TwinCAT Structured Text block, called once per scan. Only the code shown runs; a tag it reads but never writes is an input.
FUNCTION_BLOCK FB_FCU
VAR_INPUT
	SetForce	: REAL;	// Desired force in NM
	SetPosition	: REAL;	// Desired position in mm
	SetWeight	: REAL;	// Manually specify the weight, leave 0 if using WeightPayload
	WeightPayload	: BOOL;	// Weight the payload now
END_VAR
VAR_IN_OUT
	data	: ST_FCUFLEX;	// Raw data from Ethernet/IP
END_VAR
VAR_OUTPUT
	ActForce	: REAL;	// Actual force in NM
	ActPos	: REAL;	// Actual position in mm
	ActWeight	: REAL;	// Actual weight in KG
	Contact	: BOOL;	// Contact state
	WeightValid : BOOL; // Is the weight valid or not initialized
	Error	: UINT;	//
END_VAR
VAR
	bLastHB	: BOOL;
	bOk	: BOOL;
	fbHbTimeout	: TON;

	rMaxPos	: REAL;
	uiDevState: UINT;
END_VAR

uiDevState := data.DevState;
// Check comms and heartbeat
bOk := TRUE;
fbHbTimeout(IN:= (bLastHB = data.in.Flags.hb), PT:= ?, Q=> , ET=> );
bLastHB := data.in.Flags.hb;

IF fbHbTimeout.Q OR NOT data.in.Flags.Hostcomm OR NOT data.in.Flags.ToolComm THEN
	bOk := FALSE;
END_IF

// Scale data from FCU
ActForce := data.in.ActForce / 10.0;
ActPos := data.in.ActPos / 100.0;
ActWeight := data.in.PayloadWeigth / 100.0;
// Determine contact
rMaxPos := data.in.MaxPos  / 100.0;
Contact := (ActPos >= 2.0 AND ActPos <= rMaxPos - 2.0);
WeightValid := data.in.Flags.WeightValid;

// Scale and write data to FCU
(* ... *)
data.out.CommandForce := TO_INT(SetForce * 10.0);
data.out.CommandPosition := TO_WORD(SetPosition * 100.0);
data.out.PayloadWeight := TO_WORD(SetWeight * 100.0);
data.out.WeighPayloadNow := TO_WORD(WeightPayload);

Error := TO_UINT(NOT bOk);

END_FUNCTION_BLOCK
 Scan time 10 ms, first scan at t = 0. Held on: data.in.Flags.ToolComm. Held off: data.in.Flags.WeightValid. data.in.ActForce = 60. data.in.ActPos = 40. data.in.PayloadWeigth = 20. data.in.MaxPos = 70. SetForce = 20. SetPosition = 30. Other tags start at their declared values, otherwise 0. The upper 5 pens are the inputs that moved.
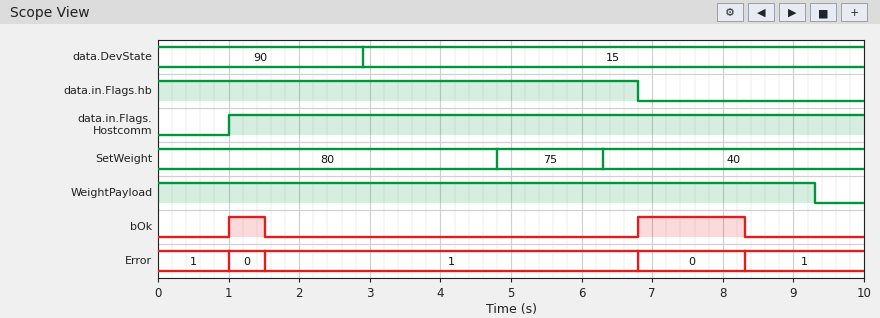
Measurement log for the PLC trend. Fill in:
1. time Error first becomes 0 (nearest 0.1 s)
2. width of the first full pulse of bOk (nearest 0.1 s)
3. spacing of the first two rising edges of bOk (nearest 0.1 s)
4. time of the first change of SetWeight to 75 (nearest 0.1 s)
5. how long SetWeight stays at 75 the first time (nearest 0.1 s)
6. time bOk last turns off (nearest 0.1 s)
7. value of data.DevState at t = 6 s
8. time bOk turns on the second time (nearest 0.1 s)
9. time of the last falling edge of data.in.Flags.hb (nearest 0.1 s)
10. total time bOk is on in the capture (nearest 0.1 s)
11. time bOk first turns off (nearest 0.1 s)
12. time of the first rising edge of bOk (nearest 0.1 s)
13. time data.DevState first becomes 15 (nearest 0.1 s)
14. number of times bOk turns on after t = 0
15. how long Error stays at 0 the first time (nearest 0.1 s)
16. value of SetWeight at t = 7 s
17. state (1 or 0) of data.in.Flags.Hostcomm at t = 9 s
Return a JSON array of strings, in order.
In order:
["1.0 s", "0.5 s", "5.8 s", "4.8 s", "1.5 s", "8.3 s", "15", "6.8 s", "6.8 s", "2.0 s", "1.5 s", "1.0 s", "2.9 s", "2", "0.5 s", "40", "1"]
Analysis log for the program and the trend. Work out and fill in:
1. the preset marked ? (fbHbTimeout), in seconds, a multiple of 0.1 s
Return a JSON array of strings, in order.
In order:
["1.5 s"]
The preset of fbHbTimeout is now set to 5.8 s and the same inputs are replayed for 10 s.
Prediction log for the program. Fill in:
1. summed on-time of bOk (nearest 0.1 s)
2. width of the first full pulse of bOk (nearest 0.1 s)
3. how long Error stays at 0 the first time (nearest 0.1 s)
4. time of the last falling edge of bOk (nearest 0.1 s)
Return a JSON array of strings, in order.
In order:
["8.0 s", "4.8 s", "4.8 s", "5.8 s"]
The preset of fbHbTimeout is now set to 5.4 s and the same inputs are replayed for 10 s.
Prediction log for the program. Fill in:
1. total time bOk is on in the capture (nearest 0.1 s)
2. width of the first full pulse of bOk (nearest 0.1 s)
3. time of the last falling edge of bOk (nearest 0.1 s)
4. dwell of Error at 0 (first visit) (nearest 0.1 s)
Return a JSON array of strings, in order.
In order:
["7.6 s", "4.4 s", "5.4 s", "4.4 s"]
